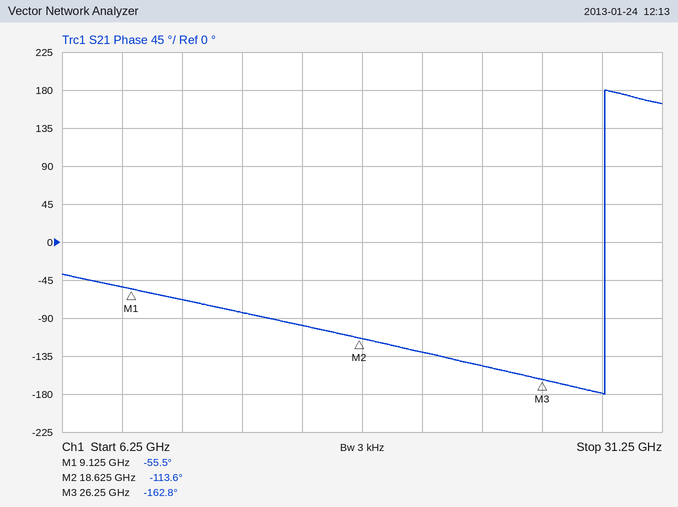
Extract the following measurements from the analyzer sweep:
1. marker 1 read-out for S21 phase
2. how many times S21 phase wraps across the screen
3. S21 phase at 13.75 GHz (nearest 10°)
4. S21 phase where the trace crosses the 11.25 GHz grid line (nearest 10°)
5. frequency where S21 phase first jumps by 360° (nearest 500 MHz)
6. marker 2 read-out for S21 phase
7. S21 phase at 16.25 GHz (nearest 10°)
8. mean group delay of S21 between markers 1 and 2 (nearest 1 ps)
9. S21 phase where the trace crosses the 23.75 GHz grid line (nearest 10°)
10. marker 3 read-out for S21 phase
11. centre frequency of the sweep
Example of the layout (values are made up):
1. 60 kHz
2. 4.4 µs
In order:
1. -55.5°
2. 1
3. -80°
4. -70°
5. 29.0 GHz
6. -113.6°
7. -100°
8. 17 ps
9. -150°
10. -162.8°
11. 18.75 GHz
